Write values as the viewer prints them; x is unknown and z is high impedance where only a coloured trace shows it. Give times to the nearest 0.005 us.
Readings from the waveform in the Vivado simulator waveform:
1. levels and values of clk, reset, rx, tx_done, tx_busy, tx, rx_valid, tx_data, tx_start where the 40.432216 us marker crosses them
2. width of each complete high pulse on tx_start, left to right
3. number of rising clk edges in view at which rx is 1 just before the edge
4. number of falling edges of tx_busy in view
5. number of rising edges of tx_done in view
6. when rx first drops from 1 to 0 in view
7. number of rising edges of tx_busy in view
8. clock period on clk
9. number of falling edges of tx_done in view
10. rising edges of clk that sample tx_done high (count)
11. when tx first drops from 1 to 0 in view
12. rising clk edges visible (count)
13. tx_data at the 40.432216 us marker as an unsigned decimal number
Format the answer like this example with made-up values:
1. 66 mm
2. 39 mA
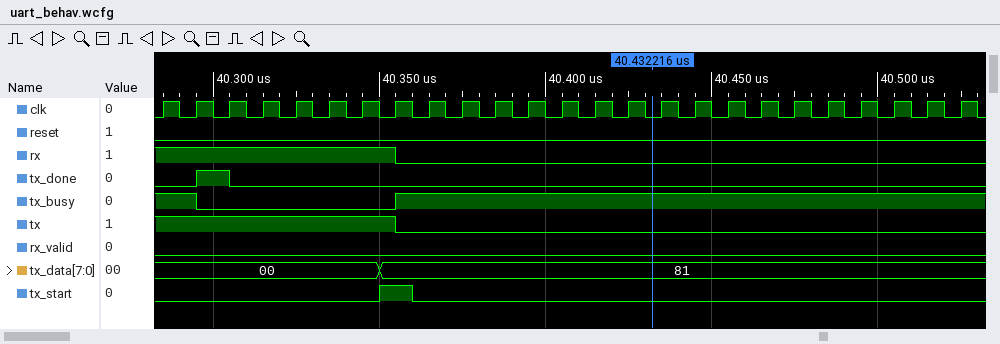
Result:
1. clk=0, reset=0, rx=0, tx_done=0, tx_busy=1, tx=0, rx_valid=0, tx_data=81, tx_start=0
2. 0.01 us
3. 8
4. 1
5. 1
6. 40.355 us
7. 1
8. 0.01 us
9. 1
10. 1
11. 40.355 us
12. 25
13. 129
